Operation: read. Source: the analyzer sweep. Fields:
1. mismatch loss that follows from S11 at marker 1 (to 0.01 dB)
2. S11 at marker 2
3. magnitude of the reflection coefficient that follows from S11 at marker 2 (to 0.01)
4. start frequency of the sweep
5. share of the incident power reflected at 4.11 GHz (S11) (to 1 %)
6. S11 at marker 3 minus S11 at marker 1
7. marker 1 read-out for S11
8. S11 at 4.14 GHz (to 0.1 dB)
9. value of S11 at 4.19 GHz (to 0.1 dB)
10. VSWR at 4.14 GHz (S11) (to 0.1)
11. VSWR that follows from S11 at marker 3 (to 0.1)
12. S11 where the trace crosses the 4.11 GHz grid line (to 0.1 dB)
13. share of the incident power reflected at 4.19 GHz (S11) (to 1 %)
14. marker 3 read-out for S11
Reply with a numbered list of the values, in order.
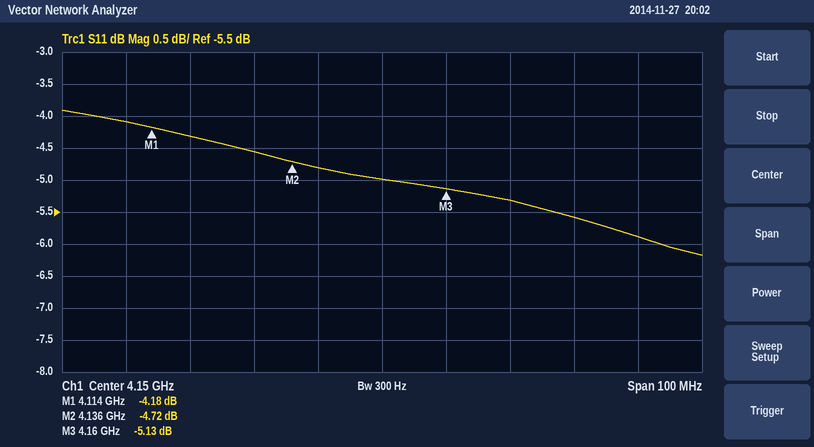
1. 2.09 dB
2. -4.72 dB
3. 0.58
4. 4.1 GHz
5. 39 %
6. -0.95 dB
7. -4.18 dB
8. -4.8 dB
9. -5.9 dB
10. 3.7
11. 3.5
12. -4.1 dB
13. 26 %
14. -5.13 dB
